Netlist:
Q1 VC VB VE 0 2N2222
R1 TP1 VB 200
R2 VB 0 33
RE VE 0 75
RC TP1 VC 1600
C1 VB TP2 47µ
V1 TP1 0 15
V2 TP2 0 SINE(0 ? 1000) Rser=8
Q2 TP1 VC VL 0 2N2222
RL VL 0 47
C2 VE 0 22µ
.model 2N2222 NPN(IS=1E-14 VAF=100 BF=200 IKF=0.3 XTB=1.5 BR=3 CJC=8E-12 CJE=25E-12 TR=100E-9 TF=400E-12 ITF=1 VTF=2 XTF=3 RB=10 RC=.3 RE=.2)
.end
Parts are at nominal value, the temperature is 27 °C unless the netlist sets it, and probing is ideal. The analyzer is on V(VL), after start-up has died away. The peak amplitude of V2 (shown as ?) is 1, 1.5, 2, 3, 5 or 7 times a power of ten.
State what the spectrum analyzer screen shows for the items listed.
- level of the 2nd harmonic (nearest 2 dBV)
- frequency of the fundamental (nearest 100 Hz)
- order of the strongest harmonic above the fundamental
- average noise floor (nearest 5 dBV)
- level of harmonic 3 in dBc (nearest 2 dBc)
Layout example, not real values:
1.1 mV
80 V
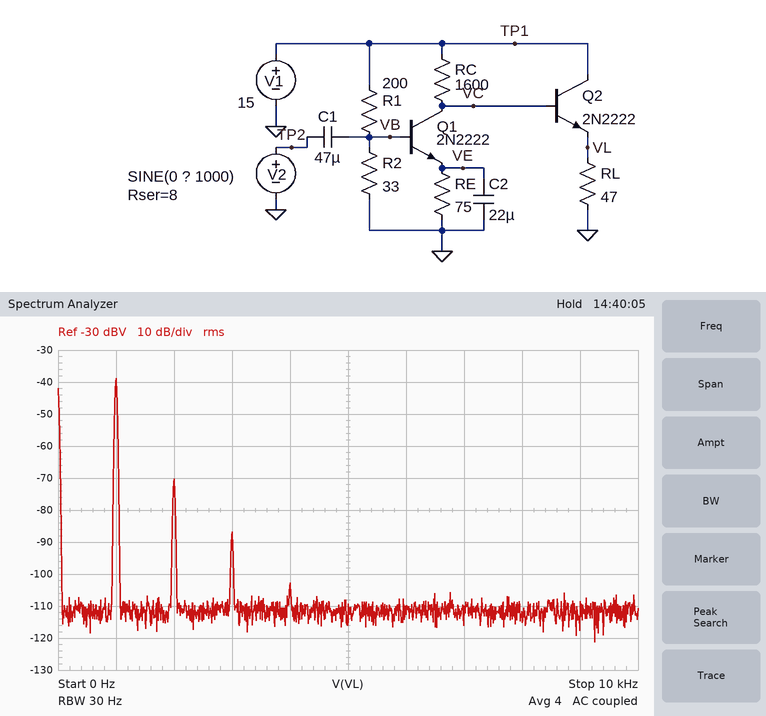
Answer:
-70 dBV
1.0 kHz
2
-110 dBV
-48 dBc
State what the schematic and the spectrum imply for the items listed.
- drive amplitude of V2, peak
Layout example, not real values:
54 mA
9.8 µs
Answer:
70 mV
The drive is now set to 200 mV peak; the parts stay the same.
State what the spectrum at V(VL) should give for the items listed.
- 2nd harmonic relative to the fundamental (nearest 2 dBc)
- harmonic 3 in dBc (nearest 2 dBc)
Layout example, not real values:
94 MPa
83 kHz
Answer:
-8 dBc
-12 dBc
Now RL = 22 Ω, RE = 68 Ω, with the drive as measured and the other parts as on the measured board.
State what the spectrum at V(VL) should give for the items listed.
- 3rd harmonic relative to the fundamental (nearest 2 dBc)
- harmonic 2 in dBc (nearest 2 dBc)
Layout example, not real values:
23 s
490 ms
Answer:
-52 dBc
-34 dBc
